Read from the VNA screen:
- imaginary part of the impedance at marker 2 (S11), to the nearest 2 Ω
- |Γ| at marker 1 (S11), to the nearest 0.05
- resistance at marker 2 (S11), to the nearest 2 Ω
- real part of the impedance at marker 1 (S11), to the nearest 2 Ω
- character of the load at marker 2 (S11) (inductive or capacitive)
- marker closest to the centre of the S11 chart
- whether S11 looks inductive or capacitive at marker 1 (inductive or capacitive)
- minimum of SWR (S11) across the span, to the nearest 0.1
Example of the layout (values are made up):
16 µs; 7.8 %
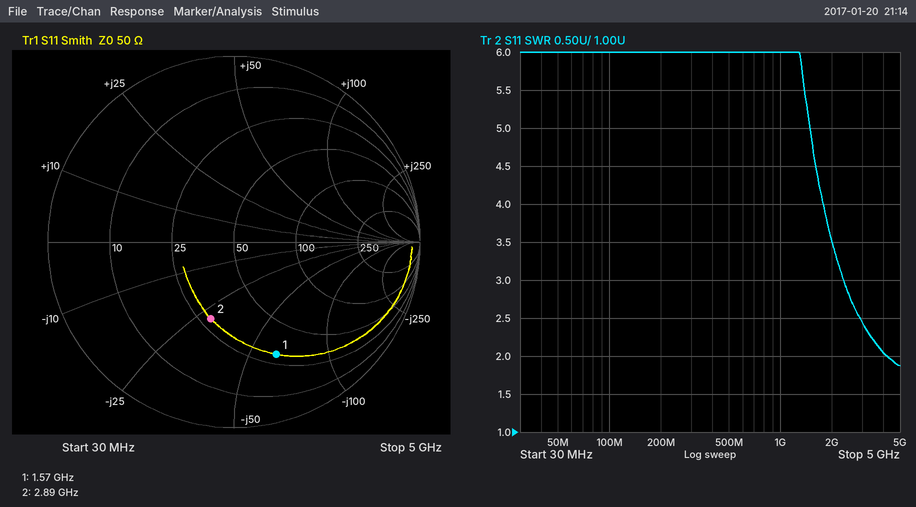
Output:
-28 Ω; 0.65; 28 Ω; 30 Ω; capacitive; marker 2; capacitive; 1.9
